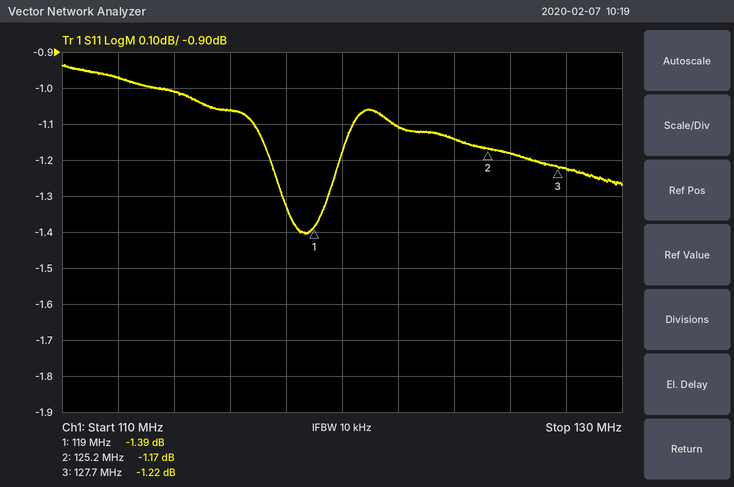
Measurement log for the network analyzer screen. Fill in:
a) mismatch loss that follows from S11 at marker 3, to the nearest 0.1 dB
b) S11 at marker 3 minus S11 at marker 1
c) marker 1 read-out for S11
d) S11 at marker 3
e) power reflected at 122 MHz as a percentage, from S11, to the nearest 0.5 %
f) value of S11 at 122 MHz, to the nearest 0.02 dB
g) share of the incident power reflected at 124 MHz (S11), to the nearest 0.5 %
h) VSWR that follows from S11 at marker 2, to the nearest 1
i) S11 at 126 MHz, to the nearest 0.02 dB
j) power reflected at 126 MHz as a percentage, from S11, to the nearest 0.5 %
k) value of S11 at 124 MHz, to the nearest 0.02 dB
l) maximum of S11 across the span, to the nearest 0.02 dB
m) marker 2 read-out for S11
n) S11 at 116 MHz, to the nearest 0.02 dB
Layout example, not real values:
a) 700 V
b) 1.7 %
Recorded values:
a) 6.1 dB
b) 0.17 dB
c) -1.39 dB
d) -1.22 dB
e) 77.5 %
f) -1.10 dB
g) 77.0 %
h) 15
i) -1.18 dB
j) 76.0 %
k) -1.14 dB
l) -0.94 dB
m) -1.17 dB
n) -1.06 dB
